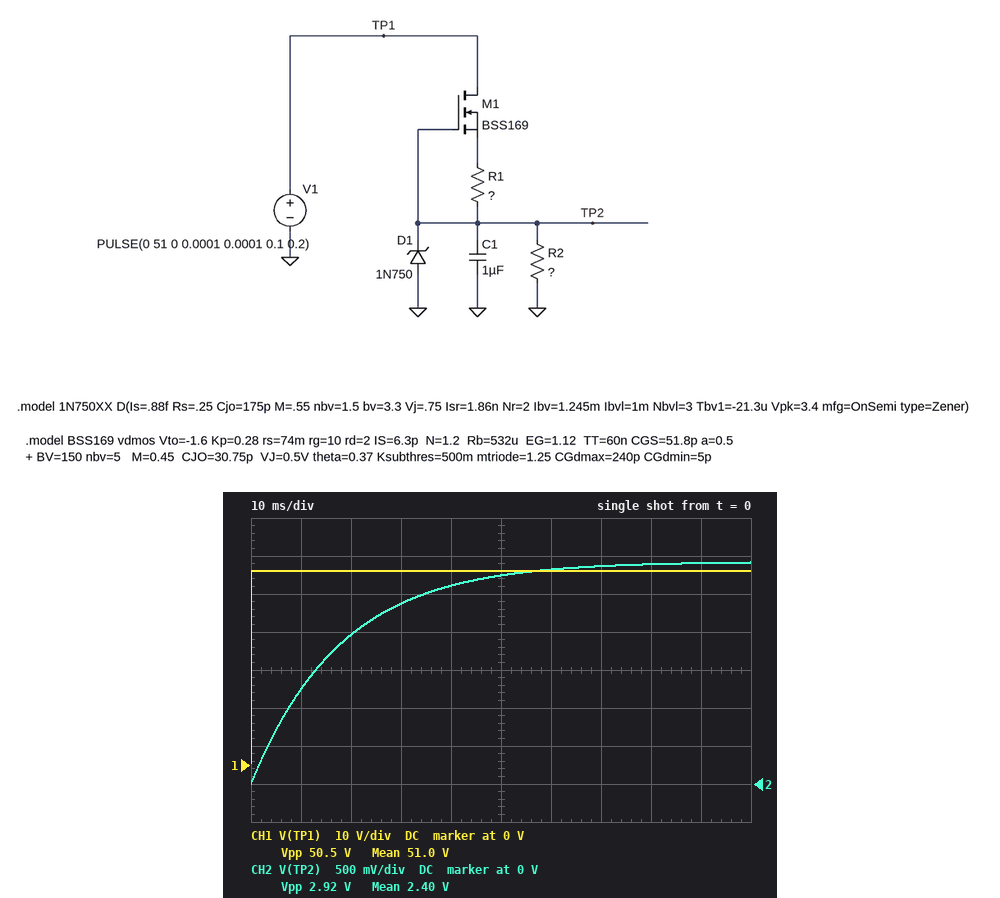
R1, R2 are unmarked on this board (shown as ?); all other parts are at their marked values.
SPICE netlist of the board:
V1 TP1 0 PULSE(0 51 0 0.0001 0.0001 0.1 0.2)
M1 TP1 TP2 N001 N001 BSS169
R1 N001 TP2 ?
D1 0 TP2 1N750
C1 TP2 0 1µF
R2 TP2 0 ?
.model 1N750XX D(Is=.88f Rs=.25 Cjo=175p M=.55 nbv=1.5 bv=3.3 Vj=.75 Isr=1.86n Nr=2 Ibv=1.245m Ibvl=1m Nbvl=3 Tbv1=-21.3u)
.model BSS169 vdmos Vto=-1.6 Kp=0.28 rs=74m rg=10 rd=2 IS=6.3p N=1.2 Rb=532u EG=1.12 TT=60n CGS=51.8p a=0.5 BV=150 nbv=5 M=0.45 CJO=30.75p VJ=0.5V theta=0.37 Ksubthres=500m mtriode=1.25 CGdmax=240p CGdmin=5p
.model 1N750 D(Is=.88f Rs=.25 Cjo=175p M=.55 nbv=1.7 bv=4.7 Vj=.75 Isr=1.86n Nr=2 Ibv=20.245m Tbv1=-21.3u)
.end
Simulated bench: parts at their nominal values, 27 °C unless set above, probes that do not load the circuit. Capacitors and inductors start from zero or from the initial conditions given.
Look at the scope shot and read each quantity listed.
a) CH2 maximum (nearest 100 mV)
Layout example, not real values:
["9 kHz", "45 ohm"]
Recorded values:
["2.9 V"]
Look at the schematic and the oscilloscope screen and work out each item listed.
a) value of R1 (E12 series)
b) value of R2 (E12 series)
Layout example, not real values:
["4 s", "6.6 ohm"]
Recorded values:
["18 kΩ", "18 kΩ"]
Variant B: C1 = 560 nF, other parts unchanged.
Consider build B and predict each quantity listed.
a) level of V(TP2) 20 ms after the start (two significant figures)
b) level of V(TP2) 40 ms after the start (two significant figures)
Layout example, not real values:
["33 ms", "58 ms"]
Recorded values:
["2.5 V", "2.9 V"]
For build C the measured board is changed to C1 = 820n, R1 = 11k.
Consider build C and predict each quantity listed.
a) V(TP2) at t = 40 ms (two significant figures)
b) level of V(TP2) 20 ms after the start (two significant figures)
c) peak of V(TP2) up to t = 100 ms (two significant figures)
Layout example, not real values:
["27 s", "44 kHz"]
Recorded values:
["4.3 V", "3.4 V", "4.4 V"]
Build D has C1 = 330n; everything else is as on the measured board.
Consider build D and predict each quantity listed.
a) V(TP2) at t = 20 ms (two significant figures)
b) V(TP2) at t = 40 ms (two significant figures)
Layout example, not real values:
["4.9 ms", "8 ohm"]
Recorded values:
["2.8 V", "2.9 V"]
